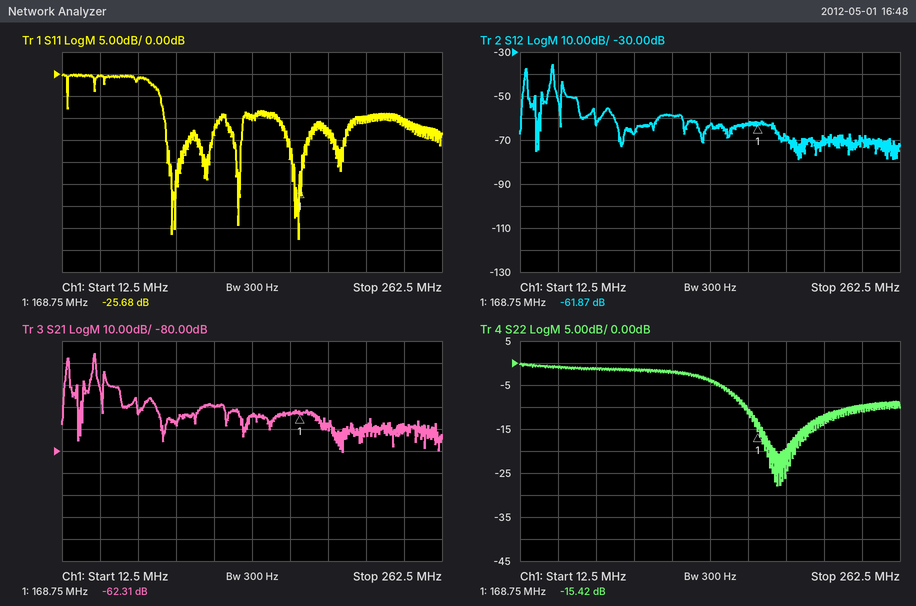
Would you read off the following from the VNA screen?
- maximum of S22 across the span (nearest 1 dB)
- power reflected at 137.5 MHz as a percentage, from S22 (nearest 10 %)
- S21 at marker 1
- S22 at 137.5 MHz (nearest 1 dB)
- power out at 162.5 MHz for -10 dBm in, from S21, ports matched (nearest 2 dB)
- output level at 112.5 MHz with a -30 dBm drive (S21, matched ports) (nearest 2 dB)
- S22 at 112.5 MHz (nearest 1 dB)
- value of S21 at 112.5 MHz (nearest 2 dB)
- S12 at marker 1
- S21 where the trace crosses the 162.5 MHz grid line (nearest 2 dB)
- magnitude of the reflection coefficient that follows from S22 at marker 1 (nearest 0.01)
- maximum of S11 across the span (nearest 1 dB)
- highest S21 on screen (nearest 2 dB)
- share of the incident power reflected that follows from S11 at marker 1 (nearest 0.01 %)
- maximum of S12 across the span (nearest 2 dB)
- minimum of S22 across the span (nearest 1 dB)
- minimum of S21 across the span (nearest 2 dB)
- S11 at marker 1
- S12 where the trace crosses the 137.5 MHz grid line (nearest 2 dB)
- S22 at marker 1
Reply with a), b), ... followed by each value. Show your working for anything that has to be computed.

a) 0 dB
b) 10^(-4/10) ≈ 40 %
c) -62.31 dB
d) -4 dB
e) -10 dBm + (-62 dB) = -72 dBm
f) -30 dBm + (-60 dB) = -90 dBm
g) -2 dB
h) -60 dB
i) -61.87 dB
j) -62 dB
k) 10^(-15.42/20) ≈ 0.17
l) 0 dB
m) -36 dB
n) 10^(-25.68/10) ≈ 0.27 %
o) -36 dB
p) -28 dB
q) -80 dB
r) -25.68 dB
s) -64 dB
t) -15.42 dB
